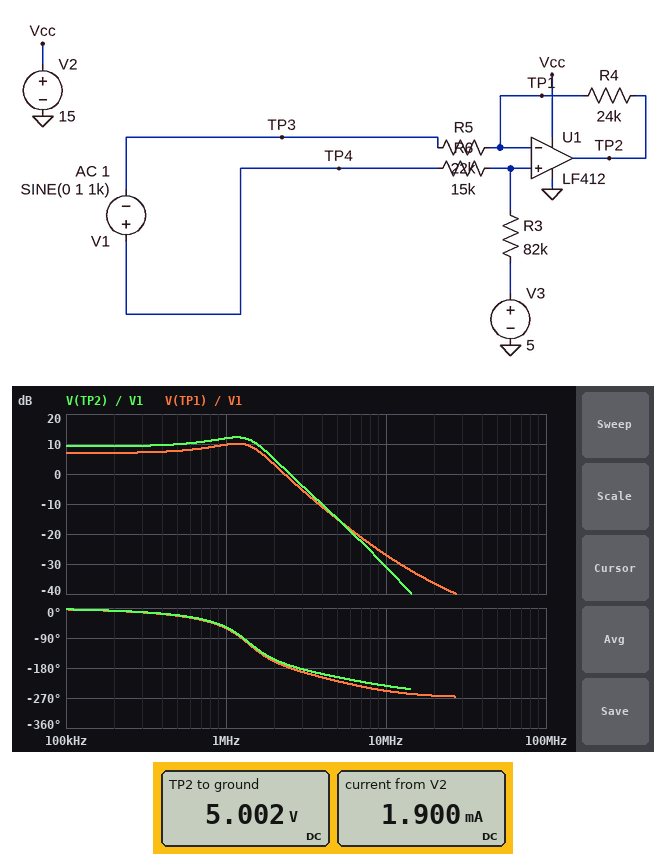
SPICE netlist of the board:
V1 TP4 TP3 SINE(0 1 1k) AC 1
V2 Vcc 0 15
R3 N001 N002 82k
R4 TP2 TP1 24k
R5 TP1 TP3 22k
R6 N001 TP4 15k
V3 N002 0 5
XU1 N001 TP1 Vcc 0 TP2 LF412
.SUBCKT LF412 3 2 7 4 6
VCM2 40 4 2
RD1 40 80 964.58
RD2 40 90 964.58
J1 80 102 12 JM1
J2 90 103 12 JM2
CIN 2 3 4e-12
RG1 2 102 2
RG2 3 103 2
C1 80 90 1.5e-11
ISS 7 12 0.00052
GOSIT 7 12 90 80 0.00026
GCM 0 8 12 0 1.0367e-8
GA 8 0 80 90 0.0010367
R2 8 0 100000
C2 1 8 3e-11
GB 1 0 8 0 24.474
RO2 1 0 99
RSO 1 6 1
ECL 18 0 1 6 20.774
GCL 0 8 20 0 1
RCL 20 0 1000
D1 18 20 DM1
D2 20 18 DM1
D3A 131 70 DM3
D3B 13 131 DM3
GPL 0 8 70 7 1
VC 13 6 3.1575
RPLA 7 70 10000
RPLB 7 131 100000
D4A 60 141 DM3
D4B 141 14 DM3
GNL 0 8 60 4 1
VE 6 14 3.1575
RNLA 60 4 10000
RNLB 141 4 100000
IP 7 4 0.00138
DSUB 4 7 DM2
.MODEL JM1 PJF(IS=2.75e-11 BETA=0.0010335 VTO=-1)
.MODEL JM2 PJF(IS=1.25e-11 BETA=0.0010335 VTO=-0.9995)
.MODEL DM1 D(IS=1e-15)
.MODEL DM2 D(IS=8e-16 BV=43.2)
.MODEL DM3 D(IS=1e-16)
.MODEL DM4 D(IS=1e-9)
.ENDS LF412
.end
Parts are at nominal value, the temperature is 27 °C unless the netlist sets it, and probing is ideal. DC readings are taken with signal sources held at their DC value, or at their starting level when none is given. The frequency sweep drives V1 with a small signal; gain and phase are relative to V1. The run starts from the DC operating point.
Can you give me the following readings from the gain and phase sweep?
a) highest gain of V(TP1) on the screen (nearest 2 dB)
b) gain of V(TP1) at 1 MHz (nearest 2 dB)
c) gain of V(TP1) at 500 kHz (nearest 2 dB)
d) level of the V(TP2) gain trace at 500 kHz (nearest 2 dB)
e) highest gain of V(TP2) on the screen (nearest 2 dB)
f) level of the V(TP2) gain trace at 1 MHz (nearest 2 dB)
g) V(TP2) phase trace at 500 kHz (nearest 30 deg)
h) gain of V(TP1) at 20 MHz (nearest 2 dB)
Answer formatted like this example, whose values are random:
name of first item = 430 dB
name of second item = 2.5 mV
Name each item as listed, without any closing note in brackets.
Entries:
highest gain of V(TP1) on the screen = 10 dB
gain of V(TP1) at 1 MHz = 10 dB
gain of V(TP1) at 500 kHz = 8 dB
level of the V(TP2) gain trace at 500 kHz = 10 dB
highest gain of V(TP2) on the screen = 12 dB
level of the V(TP2) gain trace at 1 MHz = 12 dB
V(TP2) phase trace at 500 kHz = -30 deg
gain of V(TP1) at 20 MHz = -36 dB
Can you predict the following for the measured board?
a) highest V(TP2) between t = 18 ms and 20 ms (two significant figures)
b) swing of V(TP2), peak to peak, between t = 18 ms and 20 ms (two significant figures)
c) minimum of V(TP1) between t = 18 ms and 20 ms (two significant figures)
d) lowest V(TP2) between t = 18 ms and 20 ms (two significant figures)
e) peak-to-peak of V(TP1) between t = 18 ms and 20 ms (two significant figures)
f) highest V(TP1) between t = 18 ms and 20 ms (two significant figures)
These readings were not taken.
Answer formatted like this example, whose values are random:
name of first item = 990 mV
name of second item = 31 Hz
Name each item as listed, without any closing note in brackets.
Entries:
highest V(TP2) between t = 18 ms and 20 ms = 7.9 V
swing of V(TP2), peak to peak, between t = 18 ms and 20 ms = 5.7 V
minimum of V(TP1) between t = 18 ms and 20 ms = 2.8 V
lowest V(TP2) between t = 18 ms and 20 ms = 2.2 V
peak-to-peak of V(TP1) between t = 18 ms and 20 ms = 4.4 V
highest V(TP1) between t = 18 ms and 20 ms = 7.2 V
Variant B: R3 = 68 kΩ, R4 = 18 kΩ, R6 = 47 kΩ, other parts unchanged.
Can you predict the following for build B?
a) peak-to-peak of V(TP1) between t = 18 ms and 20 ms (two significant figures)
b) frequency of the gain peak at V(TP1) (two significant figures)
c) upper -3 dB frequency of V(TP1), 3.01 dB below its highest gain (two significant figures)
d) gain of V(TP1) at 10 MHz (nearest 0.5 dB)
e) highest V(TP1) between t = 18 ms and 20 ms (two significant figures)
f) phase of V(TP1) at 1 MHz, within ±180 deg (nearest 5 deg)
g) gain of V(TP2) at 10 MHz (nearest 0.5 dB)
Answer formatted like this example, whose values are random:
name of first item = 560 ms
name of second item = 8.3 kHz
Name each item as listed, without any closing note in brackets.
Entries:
peak-to-peak of V(TP1) between t = 18 ms and 20 ms = 2.0 V
frequency of the gain peak at V(TP1) = 1.5 MHz
upper -3 dB frequency of V(TP1), 3.01 dB below its highest gain = 1.7 MHz
gain of V(TP1) at 10 MHz = -32.5 dB
highest V(TP1) between t = 18 ms and 20 ms = 6.0 V
phase of V(TP1) at 1 MHz, within ±180 deg = -35 deg
gain of V(TP2) at 10 MHz = -36.5 dB
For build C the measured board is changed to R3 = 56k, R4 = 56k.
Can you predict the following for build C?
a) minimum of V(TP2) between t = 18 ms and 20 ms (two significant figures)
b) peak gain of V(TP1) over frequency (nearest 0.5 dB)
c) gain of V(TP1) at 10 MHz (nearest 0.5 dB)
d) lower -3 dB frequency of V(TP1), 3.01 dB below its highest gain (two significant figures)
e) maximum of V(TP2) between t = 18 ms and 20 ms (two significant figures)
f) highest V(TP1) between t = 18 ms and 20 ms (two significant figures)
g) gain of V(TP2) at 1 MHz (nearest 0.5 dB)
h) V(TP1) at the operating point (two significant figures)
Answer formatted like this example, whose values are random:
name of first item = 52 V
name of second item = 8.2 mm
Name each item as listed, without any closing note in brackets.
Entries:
minimum of V(TP2) between t = 18 ms and 20 ms = 2.1 V
peak gain of V(TP1) over frequency = 7.0 dB
gain of V(TP1) at 10 MHz = -23.5 dB
lower -3 dB frequency of V(TP1), 3.01 dB below its highest gain = 340 kHz
maximum of V(TP2) between t = 18 ms and 20 ms = 8.0 V
highest V(TP1) between t = 18 ms and 20 ms = 6.5 V
gain of V(TP2) at 1 MHz = 12.5 dB
V(TP1) at the operating point = 5.0 V
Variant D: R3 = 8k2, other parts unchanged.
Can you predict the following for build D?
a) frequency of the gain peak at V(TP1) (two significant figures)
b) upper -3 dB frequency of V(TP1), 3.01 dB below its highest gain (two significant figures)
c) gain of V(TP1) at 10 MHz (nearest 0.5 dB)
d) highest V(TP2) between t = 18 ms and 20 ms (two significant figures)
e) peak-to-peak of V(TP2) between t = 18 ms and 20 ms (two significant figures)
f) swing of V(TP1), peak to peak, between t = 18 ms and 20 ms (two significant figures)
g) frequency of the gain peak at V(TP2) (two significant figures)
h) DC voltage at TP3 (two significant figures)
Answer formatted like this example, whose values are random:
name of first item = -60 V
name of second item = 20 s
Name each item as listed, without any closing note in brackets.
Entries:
frequency of the gain peak at V(TP1) = 2.3 MHz
upper -3 dB frequency of V(TP1), 3.01 dB below its highest gain = 2.9 MHz
gain of V(TP1) at 10 MHz = -21.5 dB
highest V(TP2) between t = 18 ms and 20 ms = 5.9 V
peak-to-peak of V(TP2) between t = 18 ms and 20 ms = 1.7 V
swing of V(TP1), peak to peak, between t = 18 ms and 20 ms = 440 mV
frequency of the gain peak at V(TP2) = 2.2 MHz
DC voltage at TP3 = 5.0 V
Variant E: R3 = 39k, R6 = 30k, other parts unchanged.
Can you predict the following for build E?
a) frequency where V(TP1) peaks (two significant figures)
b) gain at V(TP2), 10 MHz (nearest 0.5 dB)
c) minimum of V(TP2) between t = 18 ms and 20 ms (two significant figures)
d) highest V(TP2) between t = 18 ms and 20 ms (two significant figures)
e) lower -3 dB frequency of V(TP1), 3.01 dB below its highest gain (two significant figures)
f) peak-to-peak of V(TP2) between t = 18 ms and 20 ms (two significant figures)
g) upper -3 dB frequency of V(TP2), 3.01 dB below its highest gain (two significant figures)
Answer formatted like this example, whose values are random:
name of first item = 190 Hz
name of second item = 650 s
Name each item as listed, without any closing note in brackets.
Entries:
frequency where V(TP1) peaks = 1.7 MHz
gain at V(TP2), 10 MHz = -34.0 dB
minimum of V(TP2) between t = 18 ms and 20 ms = 3.8 V
highest V(TP2) between t = 18 ms and 20 ms = 6.2 V
lower -3 dB frequency of V(TP1), 3.01 dB below its highest gain = 1.3 MHz
peak-to-peak of V(TP2) between t = 18 ms and 20 ms = 2.4 V
upper -3 dB frequency of V(TP2), 3.01 dB below its highest gain = 2.0 MHz
